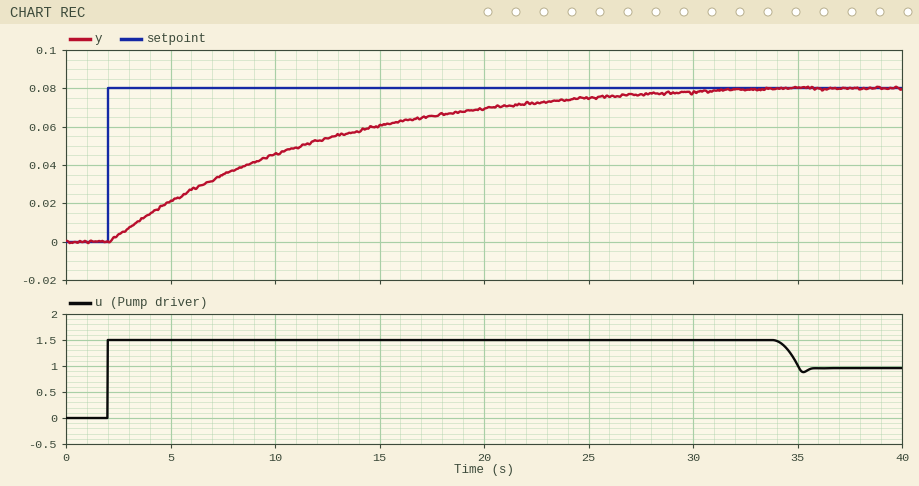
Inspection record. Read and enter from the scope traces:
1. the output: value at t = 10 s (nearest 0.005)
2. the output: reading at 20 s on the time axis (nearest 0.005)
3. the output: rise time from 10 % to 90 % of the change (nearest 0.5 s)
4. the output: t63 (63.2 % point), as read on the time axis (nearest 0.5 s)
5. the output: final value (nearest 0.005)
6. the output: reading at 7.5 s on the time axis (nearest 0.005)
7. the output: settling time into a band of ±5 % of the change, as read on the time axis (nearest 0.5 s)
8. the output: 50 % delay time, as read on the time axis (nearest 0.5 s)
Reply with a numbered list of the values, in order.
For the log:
1. 0.045
2. 0.070
3. 19.0 s
4. 11.5 s
5. 0.080
6. 0.035
7. 26.5 s
8. 8.5 s
